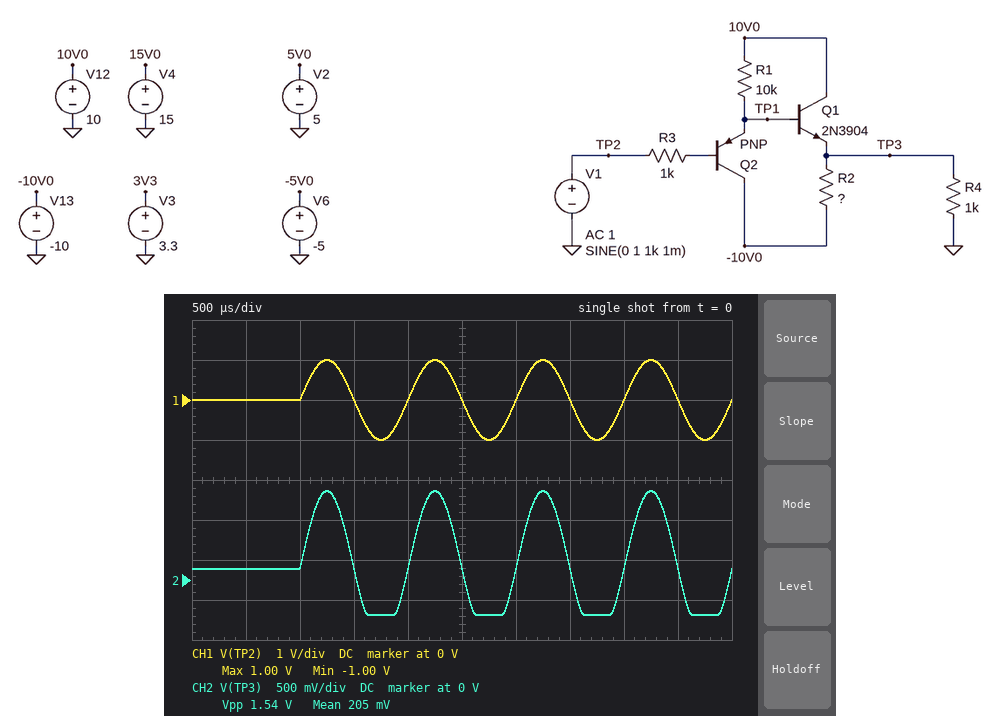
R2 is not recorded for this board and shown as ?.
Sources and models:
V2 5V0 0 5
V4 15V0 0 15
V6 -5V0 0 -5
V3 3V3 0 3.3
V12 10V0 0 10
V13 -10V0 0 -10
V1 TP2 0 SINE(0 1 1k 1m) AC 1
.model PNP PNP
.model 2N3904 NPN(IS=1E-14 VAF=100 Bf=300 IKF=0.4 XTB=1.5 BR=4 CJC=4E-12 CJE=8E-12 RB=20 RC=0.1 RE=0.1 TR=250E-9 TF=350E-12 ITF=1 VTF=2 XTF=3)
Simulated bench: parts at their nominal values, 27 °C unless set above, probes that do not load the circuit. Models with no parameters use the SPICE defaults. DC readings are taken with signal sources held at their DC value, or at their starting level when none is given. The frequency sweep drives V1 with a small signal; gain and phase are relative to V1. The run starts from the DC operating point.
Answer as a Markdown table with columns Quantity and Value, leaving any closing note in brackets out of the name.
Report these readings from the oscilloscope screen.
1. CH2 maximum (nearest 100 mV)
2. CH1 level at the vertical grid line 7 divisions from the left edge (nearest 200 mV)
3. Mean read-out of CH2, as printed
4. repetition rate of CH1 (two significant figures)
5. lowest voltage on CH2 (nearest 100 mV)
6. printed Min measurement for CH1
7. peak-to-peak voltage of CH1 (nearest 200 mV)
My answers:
| Quantity | Value |
|---|---|
| CH2 maximum | 1.1 V |
| CH1 level at the vertical grid line 7 divisions from the left edge | 0 V |
| Mean read-out of CH2, as printed | 205 mV |
| repetition rate of CH1 | 1.0 kHz |
| lowest voltage on CH2 | -400 mV |
| printed Min measurement for CH1 | -1.00 V |
| peak-to-peak voltage of CH1 | 2.0 V |
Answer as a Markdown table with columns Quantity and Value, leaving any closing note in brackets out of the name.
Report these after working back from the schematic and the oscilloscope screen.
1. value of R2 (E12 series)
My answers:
| Quantity | Value |
|---|---|
| value of R2 | 22 kΩ |
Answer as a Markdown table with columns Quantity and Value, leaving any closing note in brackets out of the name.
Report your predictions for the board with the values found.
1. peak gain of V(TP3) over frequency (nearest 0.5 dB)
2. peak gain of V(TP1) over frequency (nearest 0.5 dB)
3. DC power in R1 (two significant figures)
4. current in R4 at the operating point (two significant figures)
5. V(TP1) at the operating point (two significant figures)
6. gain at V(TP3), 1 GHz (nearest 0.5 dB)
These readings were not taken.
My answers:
| Quantity | Value |
|---|---|
| peak gain of V(TP3) over frequency | -0.5 dB |
| peak gain of V(TP1) over frequency | 0 dB |
| DC power in R1 | 8.5 mW |
| current in R4 at the operating point | 140 µA |
| V(TP1) at the operating point | 780 mV |
| gain at V(TP3), 1 GHz | -2.0 dB |
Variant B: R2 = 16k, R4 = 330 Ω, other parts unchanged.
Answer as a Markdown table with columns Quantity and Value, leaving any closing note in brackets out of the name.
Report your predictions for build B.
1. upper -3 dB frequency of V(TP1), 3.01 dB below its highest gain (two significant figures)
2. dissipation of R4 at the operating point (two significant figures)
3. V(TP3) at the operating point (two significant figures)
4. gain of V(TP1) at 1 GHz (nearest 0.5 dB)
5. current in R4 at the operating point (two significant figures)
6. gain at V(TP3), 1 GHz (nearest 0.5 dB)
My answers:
| Quantity | Value |
|---|---|
| upper -3 dB frequency of V(TP1), 3.01 dB below its highest gain | 1.7 GHz |
| dissipation of R4 at the operating point | 49 µW |
| V(TP3) at the operating point | 130 mV |
| gain of V(TP1) at 1 GHz | -2.0 dB |
| current in R4 at the operating point | 390 µA |
| gain at V(TP3), 1 GHz | -2.5 dB |
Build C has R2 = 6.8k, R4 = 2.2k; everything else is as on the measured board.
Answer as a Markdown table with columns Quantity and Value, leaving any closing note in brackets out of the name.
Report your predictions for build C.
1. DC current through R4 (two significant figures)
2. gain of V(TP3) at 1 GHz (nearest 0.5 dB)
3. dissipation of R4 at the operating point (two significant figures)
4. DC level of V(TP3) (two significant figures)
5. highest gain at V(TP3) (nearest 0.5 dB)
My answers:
| Quantity | Value |
|---|---|
| DC current through R4 | 53 µA |
| gain of V(TP3) at 1 GHz | -1.5 dB |
| dissipation of R4 at the operating point | 6.2 µW |
| DC level of V(TP3) | 120 mV |
| highest gain at V(TP3) | 0 dB |
